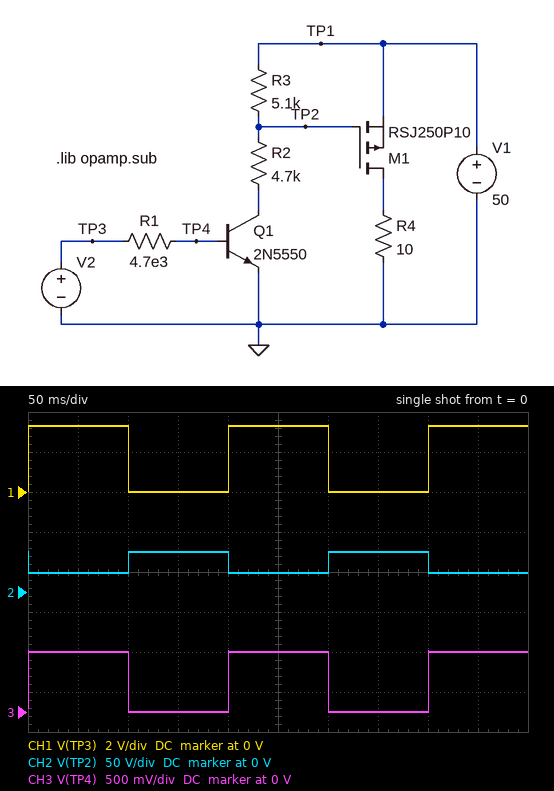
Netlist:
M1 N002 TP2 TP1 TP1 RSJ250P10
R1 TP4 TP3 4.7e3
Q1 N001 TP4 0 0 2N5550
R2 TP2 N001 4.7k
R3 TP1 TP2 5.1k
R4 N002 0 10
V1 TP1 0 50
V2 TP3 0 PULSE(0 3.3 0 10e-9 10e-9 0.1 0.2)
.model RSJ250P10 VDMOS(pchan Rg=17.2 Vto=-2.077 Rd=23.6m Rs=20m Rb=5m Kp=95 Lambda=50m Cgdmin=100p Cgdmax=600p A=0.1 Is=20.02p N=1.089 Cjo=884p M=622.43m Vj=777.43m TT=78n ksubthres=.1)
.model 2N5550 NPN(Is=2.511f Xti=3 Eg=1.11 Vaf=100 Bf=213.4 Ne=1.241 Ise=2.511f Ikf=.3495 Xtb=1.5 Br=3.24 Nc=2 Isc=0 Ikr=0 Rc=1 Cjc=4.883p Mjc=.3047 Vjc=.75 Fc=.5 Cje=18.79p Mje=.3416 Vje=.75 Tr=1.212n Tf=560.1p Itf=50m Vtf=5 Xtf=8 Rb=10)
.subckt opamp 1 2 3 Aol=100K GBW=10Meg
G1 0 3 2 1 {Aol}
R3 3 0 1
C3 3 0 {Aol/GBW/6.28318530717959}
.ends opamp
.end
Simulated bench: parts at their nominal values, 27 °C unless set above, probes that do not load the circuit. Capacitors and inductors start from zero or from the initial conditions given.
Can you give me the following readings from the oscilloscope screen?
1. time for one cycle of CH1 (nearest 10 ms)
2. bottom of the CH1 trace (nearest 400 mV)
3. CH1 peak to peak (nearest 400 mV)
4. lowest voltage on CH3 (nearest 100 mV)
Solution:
200 ms
0 V
3.2 V
0 V
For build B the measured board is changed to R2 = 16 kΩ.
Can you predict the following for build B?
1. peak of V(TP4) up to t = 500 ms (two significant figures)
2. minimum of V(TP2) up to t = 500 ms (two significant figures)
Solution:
740 mV
38 V
